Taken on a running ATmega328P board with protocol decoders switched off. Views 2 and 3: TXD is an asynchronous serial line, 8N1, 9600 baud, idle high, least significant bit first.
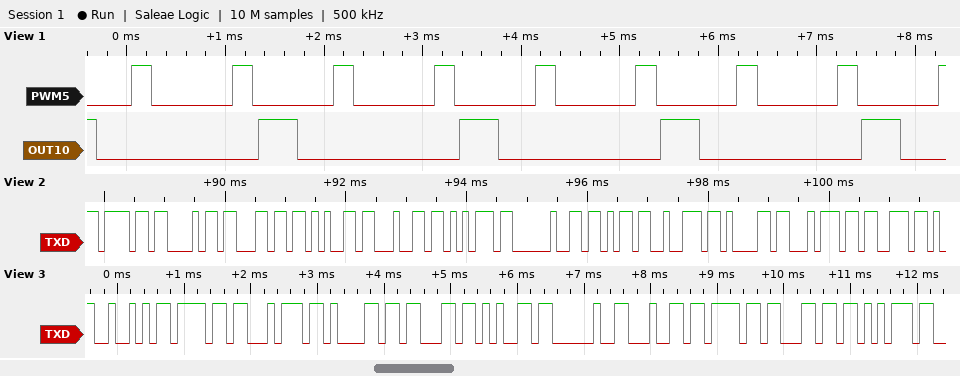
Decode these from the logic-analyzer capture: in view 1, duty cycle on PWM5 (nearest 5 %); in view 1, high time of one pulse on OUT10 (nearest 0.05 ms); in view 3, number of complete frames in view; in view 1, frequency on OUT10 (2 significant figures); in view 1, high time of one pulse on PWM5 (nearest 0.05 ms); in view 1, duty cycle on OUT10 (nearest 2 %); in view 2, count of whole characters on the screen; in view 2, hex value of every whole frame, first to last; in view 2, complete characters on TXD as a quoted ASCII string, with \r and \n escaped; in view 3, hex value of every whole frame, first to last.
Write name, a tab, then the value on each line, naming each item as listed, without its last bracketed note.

in view 1, duty cycle on PWM5	20 %
in view 1, high time of one pulse on OUT10	0.40 ms
in view 3, number of complete frames in view	11
in view 1, frequency on OUT10	490 Hz
in view 1, high time of one pulse on PWM5	0.20 ms
in view 1, duty cycle on OUT10	20 %
in view 2, count of whole characters on the screen	12
in view 2, hex value of every whole frame, first to last	0x6F 0x68 0x6C 0x65 0x64 0x75 0x20 0x6B 0x72 0x61 0x74 0x73
in view 2, complete characters on TXD as a quoted ASCII string, with \r and \n escaped	"ohledu krats"
in view 3, hex value of every whole frame, first to last	52 6F 74 61 63 65 20 64 6F 6C 75
